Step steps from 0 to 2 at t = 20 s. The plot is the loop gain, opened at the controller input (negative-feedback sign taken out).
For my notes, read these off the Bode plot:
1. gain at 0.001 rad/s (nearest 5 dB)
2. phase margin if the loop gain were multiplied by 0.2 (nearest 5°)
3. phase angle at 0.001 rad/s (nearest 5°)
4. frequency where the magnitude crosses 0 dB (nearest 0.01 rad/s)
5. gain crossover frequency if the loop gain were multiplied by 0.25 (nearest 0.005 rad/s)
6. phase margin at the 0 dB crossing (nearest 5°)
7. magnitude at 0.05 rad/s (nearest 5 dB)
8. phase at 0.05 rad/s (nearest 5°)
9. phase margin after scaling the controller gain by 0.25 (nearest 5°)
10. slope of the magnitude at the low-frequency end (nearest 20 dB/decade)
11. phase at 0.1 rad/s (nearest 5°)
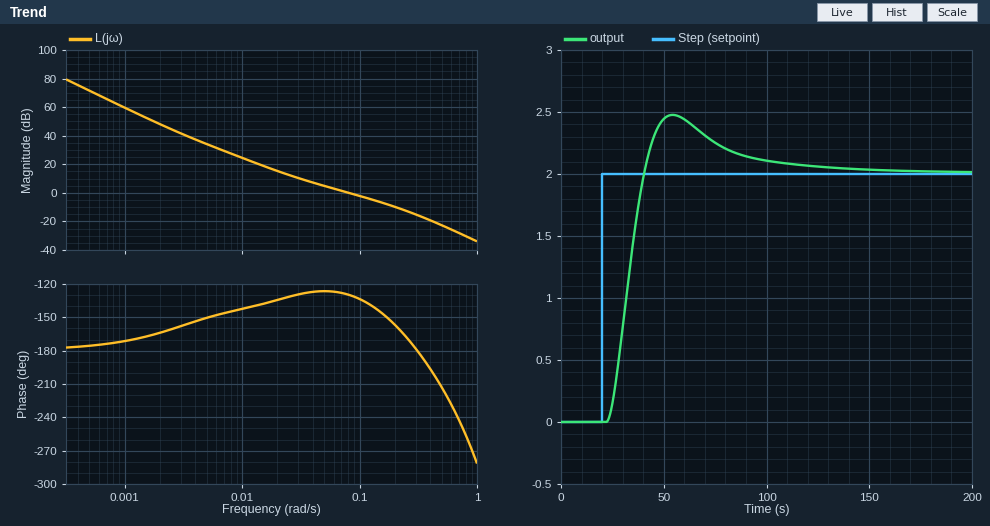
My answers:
60 dB
45°
-170°
0.08 rad/s
0.025 rad/s
50°
5 dB
-125°
50°
-40 dB/decade
-135°
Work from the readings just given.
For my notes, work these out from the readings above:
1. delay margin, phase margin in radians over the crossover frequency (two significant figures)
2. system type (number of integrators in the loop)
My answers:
11 s
2
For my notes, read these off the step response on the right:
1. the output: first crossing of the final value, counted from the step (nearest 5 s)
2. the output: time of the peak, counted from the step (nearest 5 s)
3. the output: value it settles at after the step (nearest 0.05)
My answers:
20 s
35 s
2.00
